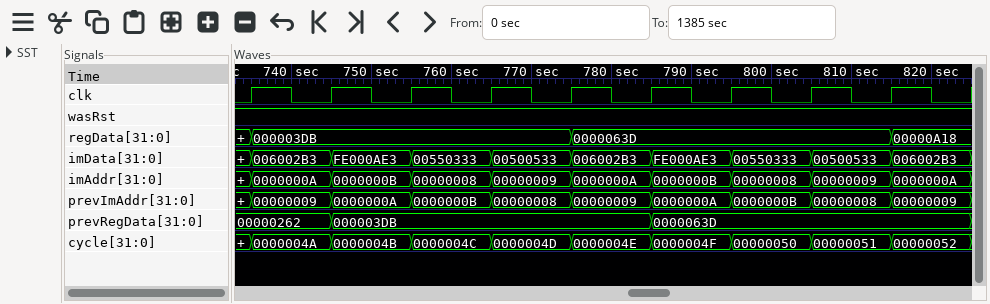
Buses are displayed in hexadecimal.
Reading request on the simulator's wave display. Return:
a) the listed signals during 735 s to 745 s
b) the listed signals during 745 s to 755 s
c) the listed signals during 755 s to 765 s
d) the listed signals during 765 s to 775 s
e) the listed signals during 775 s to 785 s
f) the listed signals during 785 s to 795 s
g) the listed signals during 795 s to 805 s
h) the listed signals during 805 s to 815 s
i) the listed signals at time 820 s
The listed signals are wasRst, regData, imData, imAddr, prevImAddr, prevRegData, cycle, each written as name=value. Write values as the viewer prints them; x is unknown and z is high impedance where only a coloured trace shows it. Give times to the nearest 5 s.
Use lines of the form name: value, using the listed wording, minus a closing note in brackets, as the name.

the listed signals during 735 s to 745 s: wasRst=1, regData=000003DB, imData=006002B3, imAddr=0000000A, prevImAddr=00000009, prevRegData=00000262, cycle=0000004A
the listed signals during 745 s to 755 s: wasRst=1, regData=000003DB, imData=FE000AE3, imAddr=0000000B, prevImAddr=0000000A, prevRegData=000003DB, cycle=0000004B
the listed signals during 755 s to 765 s: wasRst=1, regData=000003DB, imData=00550333, imAddr=00000008, prevImAddr=0000000B, prevRegData=000003DB, cycle=0000004C
the listed signals during 765 s to 775 s: wasRst=1, regData=000003DB, imData=00500533, imAddr=00000009, prevImAddr=00000008, prevRegData=000003DB, cycle=0000004D
the listed signals during 775 s to 785 s: wasRst=1, regData=0000063D, imData=006002B3, imAddr=0000000A, prevImAddr=00000009, prevRegData=000003DB, cycle=0000004E
the listed signals during 785 s to 795 s: wasRst=1, regData=0000063D, imData=FE000AE3, imAddr=0000000B, prevImAddr=0000000A, prevRegData=0000063D, cycle=0000004F
the listed signals during 795 s to 805 s: wasRst=1, regData=0000063D, imData=00550333, imAddr=00000008, prevImAddr=0000000B, prevRegData=0000063D, cycle=00000050
the listed signals during 805 s to 815 s: wasRst=1, regData=0000063D, imData=00500533, imAddr=00000009, prevImAddr=00000008, prevRegData=0000063D, cycle=00000051
the listed signals at time 820 s: wasRst=1, regData=00000A18, imData=006002B3, imAddr=0000000A, prevImAddr=00000009, prevRegData=0000063D, cycle=00000052
